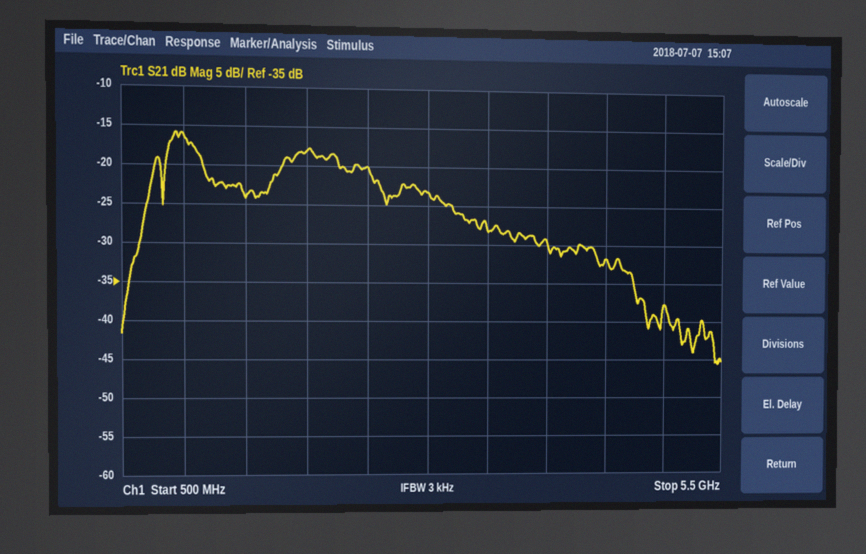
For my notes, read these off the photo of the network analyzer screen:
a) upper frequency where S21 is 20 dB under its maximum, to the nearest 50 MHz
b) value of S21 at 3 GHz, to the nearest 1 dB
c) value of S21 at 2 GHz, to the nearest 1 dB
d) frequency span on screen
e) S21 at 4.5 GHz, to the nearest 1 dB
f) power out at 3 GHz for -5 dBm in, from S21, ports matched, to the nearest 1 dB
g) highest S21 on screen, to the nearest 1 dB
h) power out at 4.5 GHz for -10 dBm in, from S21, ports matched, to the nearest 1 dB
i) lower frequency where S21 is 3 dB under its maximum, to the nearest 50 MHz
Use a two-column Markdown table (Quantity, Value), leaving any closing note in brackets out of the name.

| Quantity | Value |
|---|---|
| upper frequency where S21 is 20 dB under its maximum, to the nearest 50 MHz | 4.75 GHz |
| value of S21 at 3 GHz, to the nearest 1 dB | -23 dB |
| value of S21 at 2 GHz, to the nearest 1 dB | -18 dB |
| frequency span on screen | 5 GHz |
| S21 at 4.5 GHz, to the nearest 1 dB | -32 dB |
| power out at 3 GHz for -5 dBm in, from S21, ports matched, to the nearest 1 dB | -28 dBm |
| highest S21 on screen, to the nearest 1 dB | -16 dB |
| power out at 4.5 GHz for -10 dBm in, from S21, ports matched, to the nearest 1 dB | -42 dBm |
| lower frequency where S21 is 3 dB under its maximum, to the nearest 50 MHz | 850 MHz |
